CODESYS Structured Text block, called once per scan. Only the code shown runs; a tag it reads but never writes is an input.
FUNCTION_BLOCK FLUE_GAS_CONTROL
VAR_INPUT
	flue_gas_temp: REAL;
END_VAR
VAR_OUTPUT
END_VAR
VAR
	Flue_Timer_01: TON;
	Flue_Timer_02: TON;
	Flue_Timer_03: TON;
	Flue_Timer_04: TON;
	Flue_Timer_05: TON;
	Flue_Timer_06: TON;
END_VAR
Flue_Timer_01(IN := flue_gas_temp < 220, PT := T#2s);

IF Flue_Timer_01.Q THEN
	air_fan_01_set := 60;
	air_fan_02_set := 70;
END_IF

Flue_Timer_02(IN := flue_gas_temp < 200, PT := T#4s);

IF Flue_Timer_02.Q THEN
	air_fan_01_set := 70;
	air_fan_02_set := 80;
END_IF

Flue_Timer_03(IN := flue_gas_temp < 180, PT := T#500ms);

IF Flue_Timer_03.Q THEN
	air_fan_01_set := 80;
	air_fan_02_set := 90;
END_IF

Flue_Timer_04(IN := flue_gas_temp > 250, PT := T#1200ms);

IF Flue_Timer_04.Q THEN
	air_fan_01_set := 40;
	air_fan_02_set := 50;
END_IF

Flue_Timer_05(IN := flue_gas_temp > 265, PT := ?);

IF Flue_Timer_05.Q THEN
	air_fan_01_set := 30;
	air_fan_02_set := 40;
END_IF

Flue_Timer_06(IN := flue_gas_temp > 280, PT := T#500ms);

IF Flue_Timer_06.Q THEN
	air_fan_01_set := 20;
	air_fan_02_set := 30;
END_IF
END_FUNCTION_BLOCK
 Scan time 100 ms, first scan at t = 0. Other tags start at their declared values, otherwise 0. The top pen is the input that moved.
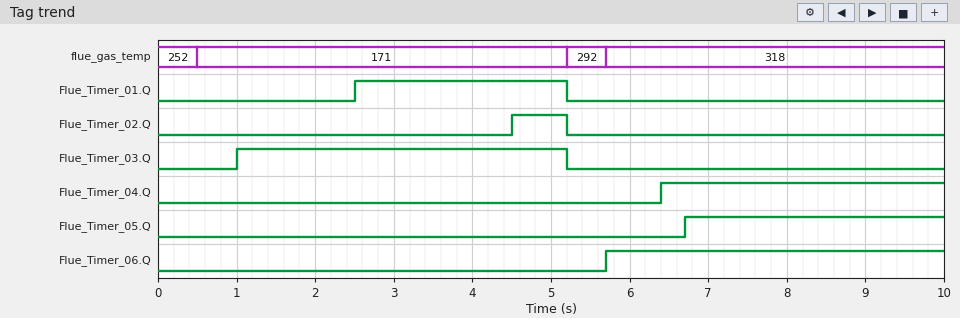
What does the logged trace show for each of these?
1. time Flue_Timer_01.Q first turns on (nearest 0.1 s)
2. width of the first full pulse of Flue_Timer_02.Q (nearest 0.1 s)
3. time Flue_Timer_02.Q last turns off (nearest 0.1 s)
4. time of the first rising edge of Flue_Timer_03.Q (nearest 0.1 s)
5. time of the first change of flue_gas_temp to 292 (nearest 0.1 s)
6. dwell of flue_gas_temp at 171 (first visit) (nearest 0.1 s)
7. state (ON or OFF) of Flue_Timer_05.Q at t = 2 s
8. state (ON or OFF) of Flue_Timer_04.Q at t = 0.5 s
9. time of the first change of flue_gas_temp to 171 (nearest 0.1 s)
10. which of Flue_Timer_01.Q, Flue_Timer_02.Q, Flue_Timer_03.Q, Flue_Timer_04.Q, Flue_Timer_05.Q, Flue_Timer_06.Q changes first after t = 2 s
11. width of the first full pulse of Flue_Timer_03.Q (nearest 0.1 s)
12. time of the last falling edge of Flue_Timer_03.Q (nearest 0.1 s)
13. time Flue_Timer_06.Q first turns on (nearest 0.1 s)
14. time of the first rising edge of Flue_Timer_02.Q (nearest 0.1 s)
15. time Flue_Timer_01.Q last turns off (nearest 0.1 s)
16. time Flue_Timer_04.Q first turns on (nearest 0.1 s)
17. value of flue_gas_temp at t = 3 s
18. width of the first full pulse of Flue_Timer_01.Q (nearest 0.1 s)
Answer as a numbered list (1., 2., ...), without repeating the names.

1. 2.5 s
2. 0.7 s
3. 5.2 s
4. 1.0 s
5. 5.2 s
6. 4.7 s
7. OFF
8. OFF
9. 0.5 s
10. Flue_Timer_01.Q
11. 4.2 s
12. 5.2 s
13. 5.7 s
14. 4.5 s
15. 5.2 s
16. 6.4 s
17. 171
18. 2.7 s
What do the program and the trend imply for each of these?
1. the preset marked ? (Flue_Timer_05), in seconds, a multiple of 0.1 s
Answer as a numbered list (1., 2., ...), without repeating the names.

1. 1.5 s
